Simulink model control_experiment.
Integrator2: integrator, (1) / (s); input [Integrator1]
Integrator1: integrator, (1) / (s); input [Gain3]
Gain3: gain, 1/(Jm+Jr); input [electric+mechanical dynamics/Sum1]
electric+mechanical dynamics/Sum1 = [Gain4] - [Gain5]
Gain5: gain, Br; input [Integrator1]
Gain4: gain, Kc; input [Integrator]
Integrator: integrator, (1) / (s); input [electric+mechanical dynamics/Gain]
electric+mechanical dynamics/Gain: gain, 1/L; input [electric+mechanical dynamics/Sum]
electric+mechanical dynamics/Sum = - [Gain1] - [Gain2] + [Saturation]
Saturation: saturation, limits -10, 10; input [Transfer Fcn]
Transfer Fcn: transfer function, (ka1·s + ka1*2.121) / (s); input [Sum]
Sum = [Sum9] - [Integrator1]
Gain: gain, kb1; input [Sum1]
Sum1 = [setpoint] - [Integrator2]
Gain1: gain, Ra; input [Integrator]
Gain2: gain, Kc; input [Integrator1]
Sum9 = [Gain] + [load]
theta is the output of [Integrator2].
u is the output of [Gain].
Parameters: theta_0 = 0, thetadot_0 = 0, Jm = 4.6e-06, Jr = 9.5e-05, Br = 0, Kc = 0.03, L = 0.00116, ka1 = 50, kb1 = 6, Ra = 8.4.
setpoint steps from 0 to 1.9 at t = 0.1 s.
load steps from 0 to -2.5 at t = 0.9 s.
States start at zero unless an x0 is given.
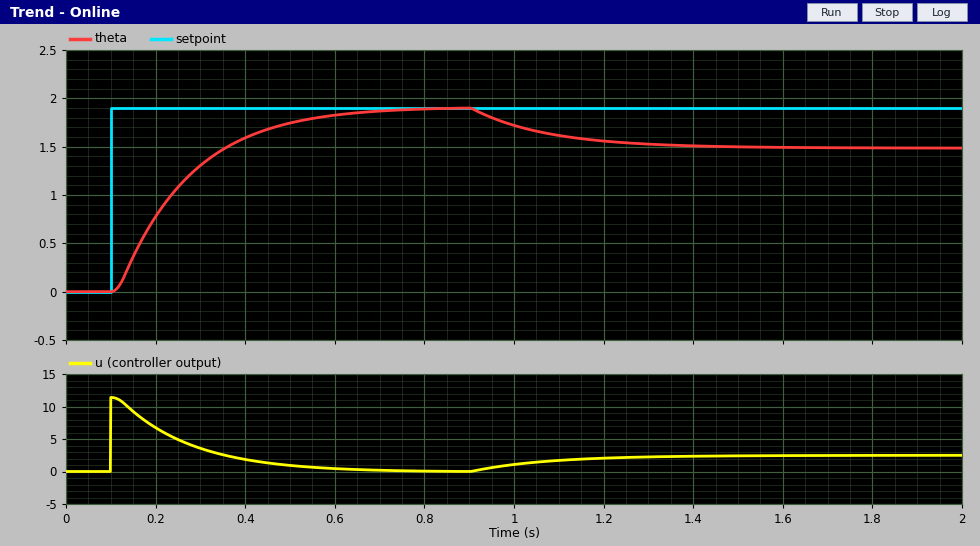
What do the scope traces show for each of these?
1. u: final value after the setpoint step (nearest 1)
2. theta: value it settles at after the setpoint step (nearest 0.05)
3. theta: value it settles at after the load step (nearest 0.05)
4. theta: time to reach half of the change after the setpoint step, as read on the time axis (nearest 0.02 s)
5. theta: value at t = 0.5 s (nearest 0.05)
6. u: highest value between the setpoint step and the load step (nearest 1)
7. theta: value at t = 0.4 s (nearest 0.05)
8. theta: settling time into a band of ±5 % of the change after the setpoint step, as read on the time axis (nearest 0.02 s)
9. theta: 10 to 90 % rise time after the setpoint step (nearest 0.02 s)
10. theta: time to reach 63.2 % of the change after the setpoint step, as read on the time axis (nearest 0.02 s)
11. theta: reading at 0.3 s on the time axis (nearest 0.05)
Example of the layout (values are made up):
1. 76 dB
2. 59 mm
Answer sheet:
1. 0
2. 1.90
3. 1.50
4. 0.22 s
5. 1.75
6. 11
7. 1.60
8. 0.56 s
9. 0.34 s
10. 0.28 s
11. 1.30
